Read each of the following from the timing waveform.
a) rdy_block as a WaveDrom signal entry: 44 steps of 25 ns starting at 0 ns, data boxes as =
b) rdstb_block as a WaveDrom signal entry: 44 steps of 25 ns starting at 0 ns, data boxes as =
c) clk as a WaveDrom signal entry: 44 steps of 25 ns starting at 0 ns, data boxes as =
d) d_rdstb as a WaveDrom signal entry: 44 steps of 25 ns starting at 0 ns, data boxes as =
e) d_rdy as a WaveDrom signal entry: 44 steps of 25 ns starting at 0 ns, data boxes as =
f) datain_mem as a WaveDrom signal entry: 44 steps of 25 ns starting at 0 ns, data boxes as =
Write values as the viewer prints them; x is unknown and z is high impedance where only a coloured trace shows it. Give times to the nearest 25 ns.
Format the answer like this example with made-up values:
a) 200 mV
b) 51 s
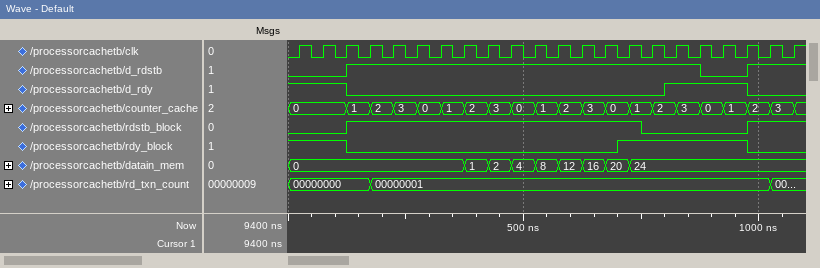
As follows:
a) {name: 'rdy_block', wave: '1....0......................1..........0....'}
b) {name: 'rdstb_block', wave: '0....1........................0........1....'}
c) {name: 'clk', wave: '01010101010101010101010101010101010101010101'}
d) {name: 'd_rdstb', wave: '0....1.............................0...1....'}
e) {name: 'd_rdy', wave: '1....0..........................1......0....'}
f) {name: 'datain_mem', wave: '=..............=.=.=.=.=.=.=.=..............', data: '0 1 2 4 8 12 16 20 24'}
